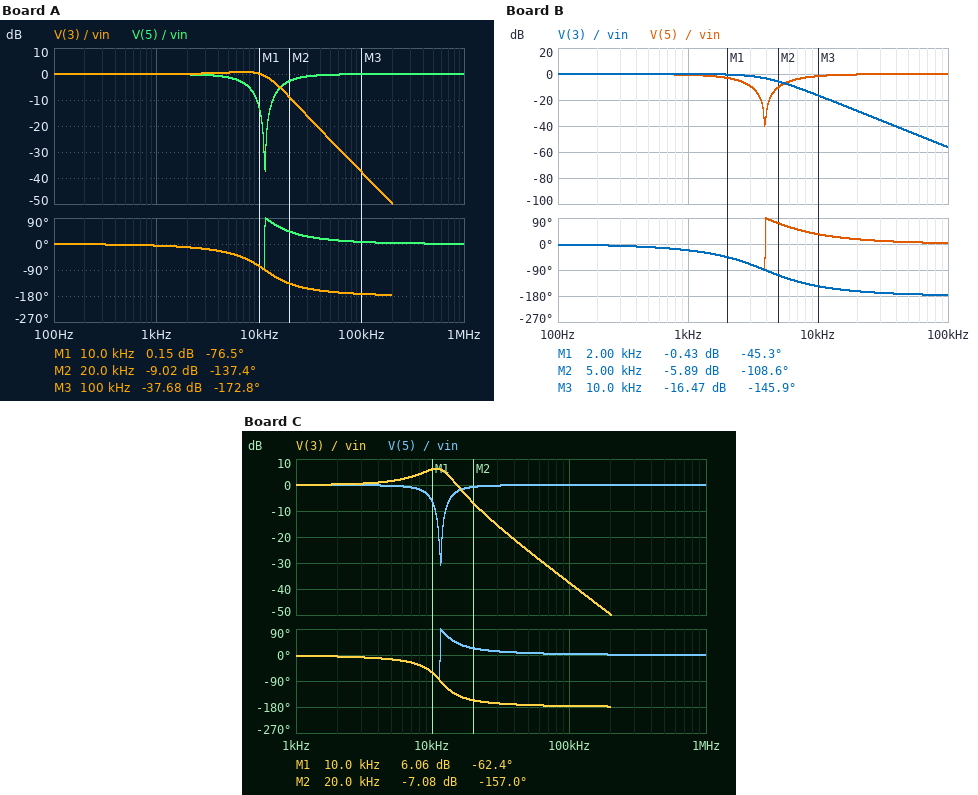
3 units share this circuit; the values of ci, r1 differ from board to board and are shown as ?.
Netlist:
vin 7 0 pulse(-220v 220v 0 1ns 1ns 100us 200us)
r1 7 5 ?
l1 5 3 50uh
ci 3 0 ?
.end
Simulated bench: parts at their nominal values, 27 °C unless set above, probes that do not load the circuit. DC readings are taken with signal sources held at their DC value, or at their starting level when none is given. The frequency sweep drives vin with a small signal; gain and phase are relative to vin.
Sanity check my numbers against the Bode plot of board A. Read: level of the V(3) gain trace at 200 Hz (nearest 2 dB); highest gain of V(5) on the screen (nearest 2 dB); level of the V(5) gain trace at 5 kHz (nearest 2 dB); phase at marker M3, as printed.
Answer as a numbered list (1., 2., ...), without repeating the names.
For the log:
1. 0 dB
2. 0 dB
3. -2 dB
4. -172.8 deg
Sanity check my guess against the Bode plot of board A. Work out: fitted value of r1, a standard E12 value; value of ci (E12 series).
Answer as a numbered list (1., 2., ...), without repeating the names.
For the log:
1. 3.9 Ω
2. 3.9 µF
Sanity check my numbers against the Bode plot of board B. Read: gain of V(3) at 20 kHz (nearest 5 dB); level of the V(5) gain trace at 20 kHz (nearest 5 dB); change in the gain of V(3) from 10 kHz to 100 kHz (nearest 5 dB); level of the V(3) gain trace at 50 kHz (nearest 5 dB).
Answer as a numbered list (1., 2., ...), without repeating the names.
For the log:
1. -30 dB
2. 0 dB
3. -40 dB
4. -45 dB
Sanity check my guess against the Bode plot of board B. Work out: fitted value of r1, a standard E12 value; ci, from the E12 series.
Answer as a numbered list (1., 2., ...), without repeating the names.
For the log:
1. 1.8 Ω
2. 33 µF
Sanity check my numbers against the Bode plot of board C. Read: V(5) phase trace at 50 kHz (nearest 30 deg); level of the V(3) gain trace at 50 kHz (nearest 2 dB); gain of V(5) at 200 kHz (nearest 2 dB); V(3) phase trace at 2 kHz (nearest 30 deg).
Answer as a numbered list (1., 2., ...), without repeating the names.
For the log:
1. 0 deg
2. -26 dB
3. 0 dB
4. 0 deg
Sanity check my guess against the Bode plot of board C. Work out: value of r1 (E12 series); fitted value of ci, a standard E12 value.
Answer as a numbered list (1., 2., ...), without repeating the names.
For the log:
1. 1.8 Ω
2. 3.9 µF
